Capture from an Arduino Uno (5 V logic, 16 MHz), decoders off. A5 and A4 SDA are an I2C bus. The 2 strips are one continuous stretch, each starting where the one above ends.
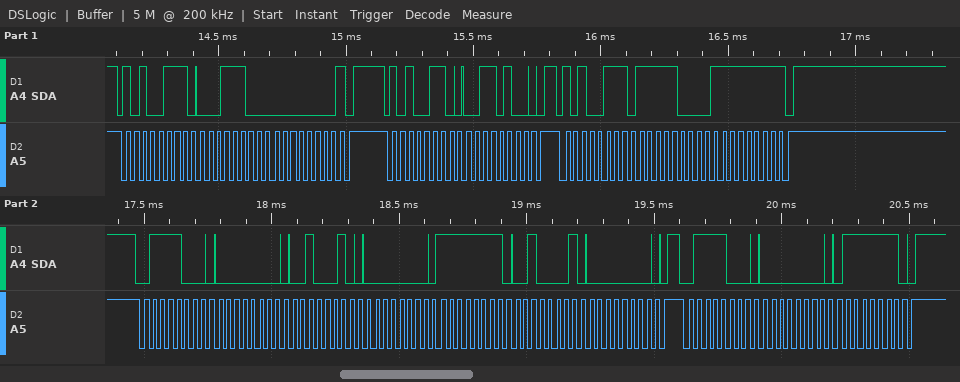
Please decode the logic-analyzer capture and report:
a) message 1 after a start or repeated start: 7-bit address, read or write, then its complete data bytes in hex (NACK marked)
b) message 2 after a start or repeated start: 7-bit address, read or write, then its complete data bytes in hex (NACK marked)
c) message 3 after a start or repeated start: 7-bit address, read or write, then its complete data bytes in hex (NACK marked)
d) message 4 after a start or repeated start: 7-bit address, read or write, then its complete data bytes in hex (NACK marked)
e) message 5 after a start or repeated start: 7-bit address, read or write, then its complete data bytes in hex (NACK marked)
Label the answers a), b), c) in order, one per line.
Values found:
a) 0x53 read: 1C 00 NACK
b) 0x53 write: 34
c) 0x53 read: F8 FF NACK
d) 0x3C write: 00 22 00 FF 21 00
e) 0x3C write: 00 7F
